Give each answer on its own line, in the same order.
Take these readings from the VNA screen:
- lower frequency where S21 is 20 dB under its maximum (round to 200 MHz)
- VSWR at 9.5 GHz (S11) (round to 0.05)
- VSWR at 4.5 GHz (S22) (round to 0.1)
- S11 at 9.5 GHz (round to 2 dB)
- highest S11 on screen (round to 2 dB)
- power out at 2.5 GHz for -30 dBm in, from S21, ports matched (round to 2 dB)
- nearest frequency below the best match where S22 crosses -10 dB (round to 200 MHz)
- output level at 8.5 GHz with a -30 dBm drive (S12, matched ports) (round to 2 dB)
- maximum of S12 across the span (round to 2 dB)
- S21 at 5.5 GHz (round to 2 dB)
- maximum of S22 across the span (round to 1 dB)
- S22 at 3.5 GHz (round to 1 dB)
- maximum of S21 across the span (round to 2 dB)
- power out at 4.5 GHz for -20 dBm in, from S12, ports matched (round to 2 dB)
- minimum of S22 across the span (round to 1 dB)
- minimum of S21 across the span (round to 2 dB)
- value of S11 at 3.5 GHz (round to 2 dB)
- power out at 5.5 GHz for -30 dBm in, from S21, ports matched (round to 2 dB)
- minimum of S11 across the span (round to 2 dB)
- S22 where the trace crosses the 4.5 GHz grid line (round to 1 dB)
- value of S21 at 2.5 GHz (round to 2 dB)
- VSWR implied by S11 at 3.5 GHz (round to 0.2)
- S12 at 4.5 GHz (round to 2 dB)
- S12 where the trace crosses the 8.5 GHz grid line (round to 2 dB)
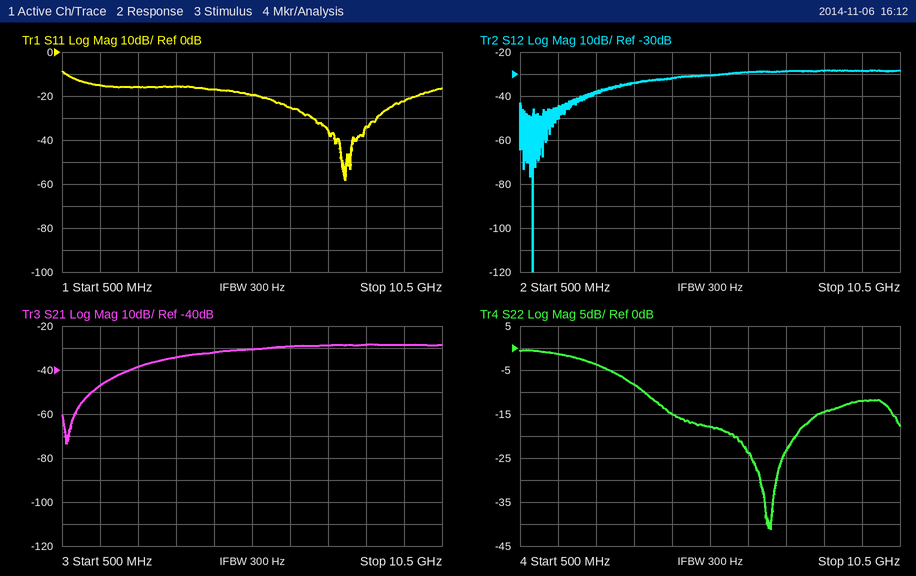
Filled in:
1.4 GHz
1.15
1.4
-22 dB
-8 dB
-68 dBm
3.8 GHz
-58 dBm
-28 dB
-30 dB
0 dB
-8 dB
-28 dB
-52 dBm
-41 dB
-74 dB
-16 dB
-60 dBm
-58 dB
-15 dB
-38 dB
1.4
-32 dB
-28 dB
